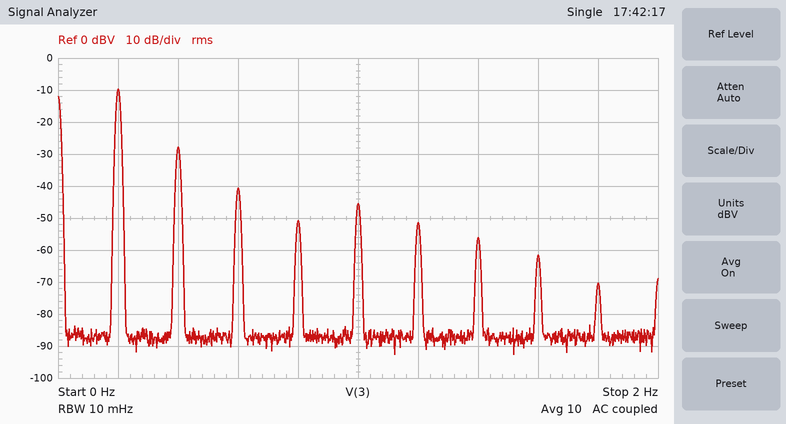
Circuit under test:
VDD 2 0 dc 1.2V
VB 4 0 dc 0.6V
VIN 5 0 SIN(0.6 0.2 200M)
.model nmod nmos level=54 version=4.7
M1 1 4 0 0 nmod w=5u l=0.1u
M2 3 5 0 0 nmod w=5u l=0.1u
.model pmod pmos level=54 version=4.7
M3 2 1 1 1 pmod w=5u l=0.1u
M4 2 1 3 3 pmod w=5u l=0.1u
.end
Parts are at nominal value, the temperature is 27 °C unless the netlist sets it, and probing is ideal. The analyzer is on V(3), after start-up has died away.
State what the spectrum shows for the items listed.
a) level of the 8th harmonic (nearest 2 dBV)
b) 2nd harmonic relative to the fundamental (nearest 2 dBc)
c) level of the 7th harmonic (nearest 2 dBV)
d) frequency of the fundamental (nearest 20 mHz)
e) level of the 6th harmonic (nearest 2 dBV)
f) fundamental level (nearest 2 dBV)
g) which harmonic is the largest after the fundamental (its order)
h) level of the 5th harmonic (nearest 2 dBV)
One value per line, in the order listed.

-62 dBV
-18 dBc
-56 dBV
200 mHz
-52 dBV
-10 dBV
2
-46 dBV
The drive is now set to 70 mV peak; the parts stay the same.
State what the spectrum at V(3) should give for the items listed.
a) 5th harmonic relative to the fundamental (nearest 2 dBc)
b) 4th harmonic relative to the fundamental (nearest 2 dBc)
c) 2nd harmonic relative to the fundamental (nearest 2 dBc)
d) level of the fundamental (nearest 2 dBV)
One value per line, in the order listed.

-58 dBc
-52 dBc
-30 dBc
-18 dBV
